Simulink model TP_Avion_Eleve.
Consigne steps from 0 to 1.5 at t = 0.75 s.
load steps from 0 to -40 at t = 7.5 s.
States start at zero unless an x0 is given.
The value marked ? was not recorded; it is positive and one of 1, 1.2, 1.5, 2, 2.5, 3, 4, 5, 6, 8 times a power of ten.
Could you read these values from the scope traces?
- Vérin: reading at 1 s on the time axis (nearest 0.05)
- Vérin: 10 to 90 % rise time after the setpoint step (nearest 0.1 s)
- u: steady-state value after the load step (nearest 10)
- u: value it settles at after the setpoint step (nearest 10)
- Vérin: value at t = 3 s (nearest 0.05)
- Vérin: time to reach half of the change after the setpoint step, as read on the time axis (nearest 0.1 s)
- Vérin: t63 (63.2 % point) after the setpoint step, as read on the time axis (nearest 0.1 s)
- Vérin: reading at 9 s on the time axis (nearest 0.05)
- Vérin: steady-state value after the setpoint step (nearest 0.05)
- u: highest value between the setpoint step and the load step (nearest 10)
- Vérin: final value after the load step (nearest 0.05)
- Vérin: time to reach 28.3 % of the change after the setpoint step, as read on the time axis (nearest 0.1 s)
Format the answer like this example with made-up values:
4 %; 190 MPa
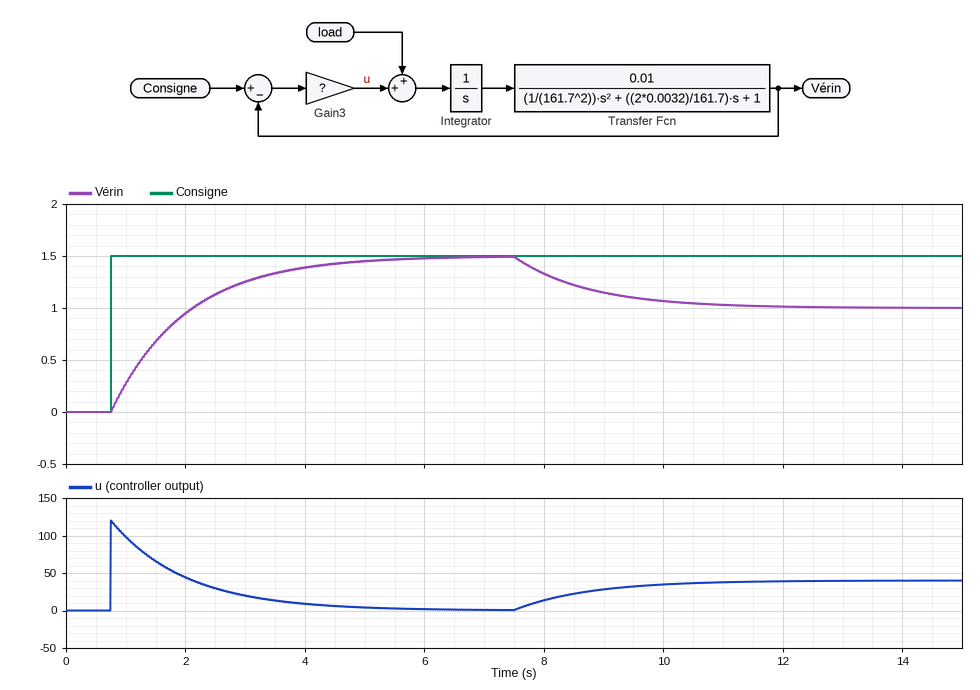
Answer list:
0.25; 2.7 s; 40; 0; 1.25; 1.6 s; 2.0 s; 1.15; 1.50; 120; 1.00; 1.2 s
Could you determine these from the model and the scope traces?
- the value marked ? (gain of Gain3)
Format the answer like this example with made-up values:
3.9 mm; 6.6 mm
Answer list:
80
